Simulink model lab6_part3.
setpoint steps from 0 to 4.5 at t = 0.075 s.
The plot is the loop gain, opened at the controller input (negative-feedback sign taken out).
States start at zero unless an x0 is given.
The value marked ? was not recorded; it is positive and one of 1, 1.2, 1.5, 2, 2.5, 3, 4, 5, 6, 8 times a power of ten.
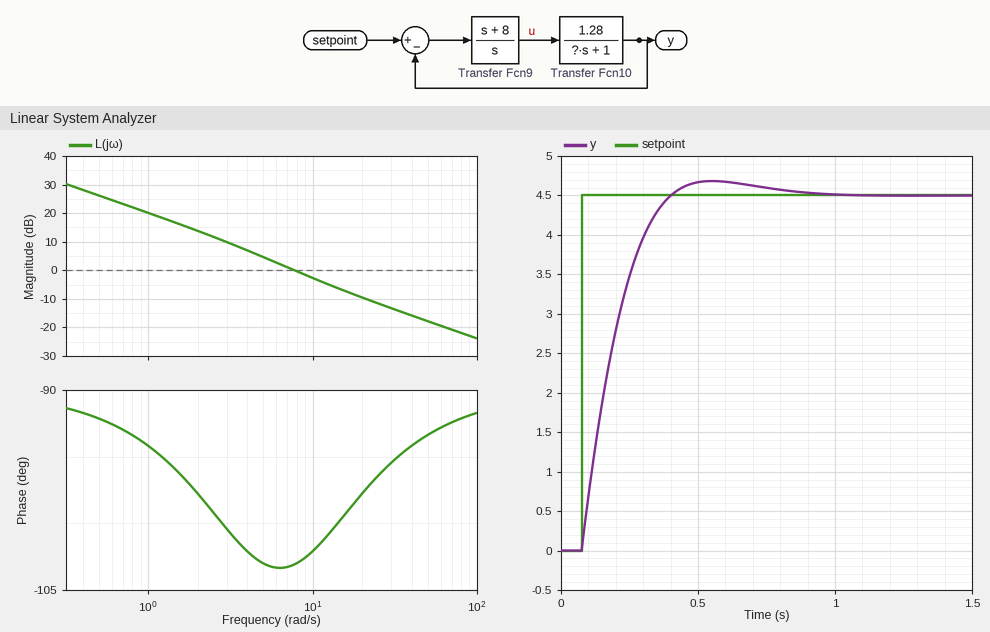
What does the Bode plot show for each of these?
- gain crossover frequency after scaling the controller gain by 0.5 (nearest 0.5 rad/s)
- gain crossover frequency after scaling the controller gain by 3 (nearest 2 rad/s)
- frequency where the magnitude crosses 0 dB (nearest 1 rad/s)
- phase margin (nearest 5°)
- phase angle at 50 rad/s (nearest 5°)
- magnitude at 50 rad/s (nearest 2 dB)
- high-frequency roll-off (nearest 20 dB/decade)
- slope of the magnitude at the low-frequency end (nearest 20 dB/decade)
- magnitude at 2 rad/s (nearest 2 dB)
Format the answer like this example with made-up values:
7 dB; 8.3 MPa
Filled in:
4.5 rad/s; 20 rad/s; 8 rad/s; 75°; -95°; -18 dB; -20 dB/decade; -20 dB/decade; 14 dB
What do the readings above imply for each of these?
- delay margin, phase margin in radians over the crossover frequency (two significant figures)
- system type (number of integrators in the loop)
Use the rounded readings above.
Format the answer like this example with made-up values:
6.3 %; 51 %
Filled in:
0.16 s; 1
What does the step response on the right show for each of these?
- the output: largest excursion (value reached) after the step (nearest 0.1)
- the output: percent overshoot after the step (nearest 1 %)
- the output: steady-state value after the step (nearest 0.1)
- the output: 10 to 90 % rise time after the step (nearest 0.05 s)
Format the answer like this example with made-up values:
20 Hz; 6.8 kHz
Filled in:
4.7; 4 %; 4.5; 0.20 s
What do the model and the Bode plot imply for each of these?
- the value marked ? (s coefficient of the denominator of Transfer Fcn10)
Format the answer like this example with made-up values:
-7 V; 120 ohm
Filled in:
0.2
